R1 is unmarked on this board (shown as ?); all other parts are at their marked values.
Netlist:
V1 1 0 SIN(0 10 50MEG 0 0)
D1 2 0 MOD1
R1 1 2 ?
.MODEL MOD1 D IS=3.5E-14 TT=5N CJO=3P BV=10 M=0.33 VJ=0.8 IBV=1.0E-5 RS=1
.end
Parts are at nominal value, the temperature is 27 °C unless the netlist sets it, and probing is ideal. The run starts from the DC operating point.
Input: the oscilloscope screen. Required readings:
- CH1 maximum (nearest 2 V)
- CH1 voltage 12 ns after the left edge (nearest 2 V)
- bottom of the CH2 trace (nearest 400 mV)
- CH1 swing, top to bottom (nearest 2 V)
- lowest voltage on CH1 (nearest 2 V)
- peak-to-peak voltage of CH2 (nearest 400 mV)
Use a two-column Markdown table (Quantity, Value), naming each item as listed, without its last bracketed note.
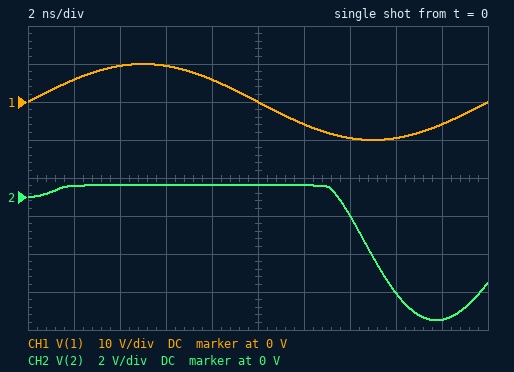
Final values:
| Quantity | Value |
|---|---|
| CH1 maximum | 10 V |
| CH1 voltage 12 ns after the left edge | -6 V |
| bottom of the CH2 trace | -6.4 V |
| CH1 swing, top to bottom | 20 V |
| lowest voltage on CH1 | -10 V |
| peak-to-peak voltage of CH2 | 7.2 V |
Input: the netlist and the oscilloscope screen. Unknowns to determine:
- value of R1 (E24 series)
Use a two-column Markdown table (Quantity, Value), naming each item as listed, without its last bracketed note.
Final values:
| Quantity | Value |
|---|---|
| value of R1 | 1.8 kΩ |
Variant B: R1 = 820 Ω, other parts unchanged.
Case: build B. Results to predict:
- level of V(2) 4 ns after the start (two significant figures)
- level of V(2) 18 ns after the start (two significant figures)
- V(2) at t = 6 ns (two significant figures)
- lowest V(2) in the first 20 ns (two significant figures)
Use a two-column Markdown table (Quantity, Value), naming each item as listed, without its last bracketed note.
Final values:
| Quantity | Value |
|---|---|
| level of V(2) 4 ns after the start | 670 mV |
| level of V(2) 18 ns after the start | -7.6 V |
| V(2) at t = 6 ns | 680 mV |
| lowest V(2) in the first 20 ns | -8.8 V |
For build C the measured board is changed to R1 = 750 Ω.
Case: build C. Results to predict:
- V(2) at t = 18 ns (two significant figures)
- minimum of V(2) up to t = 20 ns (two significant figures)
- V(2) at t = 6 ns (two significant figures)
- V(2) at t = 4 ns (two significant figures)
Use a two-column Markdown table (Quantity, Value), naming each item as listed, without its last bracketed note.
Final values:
| Quantity | Value |
|---|---|
| V(2) at t = 18 ns | -7.6 V |
| minimum of V(2) up to t = 20 ns | -9.0 V |
| V(2) at t = 6 ns | 680 mV |
| V(2) at t = 4 ns | 670 mV |
